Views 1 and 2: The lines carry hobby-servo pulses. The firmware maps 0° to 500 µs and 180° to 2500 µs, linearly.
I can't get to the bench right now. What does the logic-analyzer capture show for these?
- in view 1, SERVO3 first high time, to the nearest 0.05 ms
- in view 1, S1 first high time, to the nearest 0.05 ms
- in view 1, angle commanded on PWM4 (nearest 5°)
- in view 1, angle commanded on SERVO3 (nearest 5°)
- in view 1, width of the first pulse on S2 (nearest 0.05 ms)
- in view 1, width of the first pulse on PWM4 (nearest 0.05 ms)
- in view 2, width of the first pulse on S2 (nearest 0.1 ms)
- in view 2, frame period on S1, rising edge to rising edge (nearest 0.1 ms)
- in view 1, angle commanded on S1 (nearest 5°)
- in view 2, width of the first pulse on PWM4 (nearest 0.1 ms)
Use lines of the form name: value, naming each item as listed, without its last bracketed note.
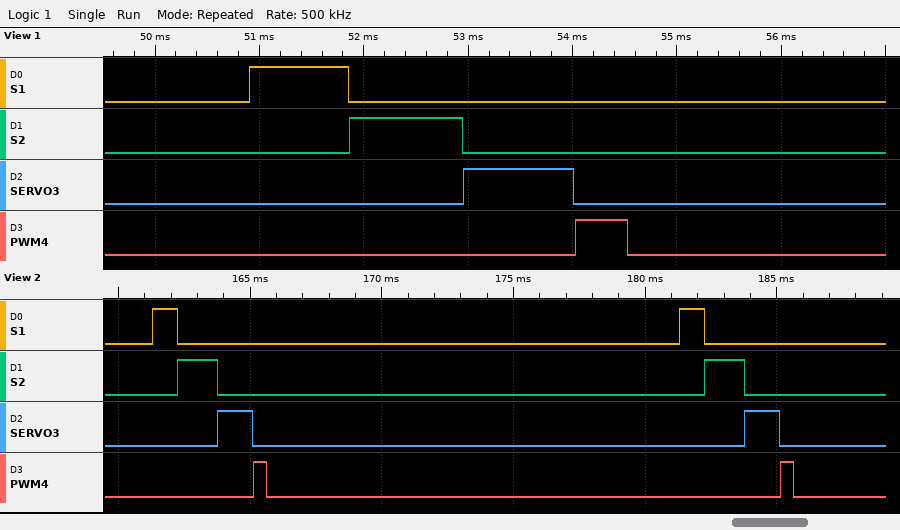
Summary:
in view 1, SERVO3 first high time, to the nearest 0.05 ms: 1.05 ms
in view 1, S1 first high time, to the nearest 0.05 ms: 0.95 ms
in view 1, angle commanded on PWM4: 0°
in view 1, angle commanded on SERVO3: 50°
in view 1, width of the first pulse on S2: 1.10 ms
in view 1, width of the first pulse on PWM4: 0.50 ms
in view 2, width of the first pulse on S2: 1.5 ms
in view 2, frame period on S1, rising edge to rising edge: 20.0 ms
in view 1, angle commanded on S1: 40°
in view 2, width of the first pulse on PWM4: 0.5 ms
